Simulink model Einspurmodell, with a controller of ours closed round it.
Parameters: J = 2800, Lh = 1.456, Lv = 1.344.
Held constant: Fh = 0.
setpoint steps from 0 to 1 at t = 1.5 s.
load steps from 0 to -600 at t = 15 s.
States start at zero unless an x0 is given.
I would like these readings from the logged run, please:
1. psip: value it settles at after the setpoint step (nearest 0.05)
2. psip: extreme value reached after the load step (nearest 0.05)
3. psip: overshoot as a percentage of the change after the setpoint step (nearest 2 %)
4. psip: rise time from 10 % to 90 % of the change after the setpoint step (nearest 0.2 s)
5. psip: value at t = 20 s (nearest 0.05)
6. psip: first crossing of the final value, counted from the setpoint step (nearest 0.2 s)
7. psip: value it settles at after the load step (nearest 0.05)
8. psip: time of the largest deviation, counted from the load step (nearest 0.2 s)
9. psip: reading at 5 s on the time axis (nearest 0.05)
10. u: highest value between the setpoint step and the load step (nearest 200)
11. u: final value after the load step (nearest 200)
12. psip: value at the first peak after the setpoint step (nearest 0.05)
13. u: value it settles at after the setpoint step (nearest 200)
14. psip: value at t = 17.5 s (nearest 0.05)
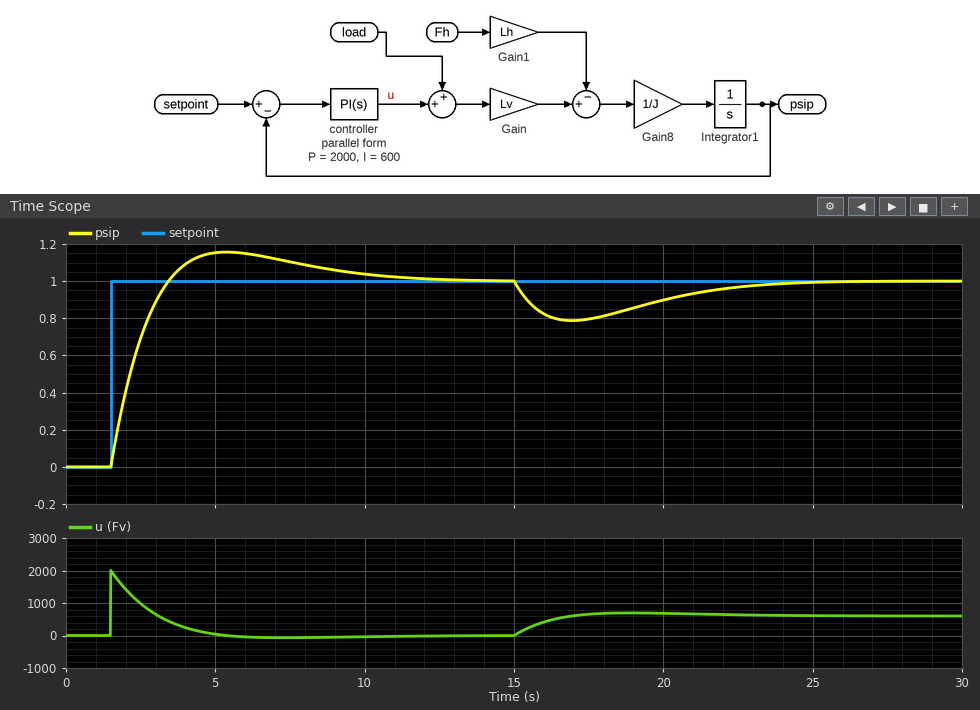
1.00
0.80
16 %
1.4 s
0.90
2.0 s
1.00
2.0 s
1.15
2000
600
1.15
0
0.80
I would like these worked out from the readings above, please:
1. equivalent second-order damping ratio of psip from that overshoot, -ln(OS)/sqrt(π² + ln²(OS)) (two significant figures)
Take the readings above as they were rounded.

0.50
